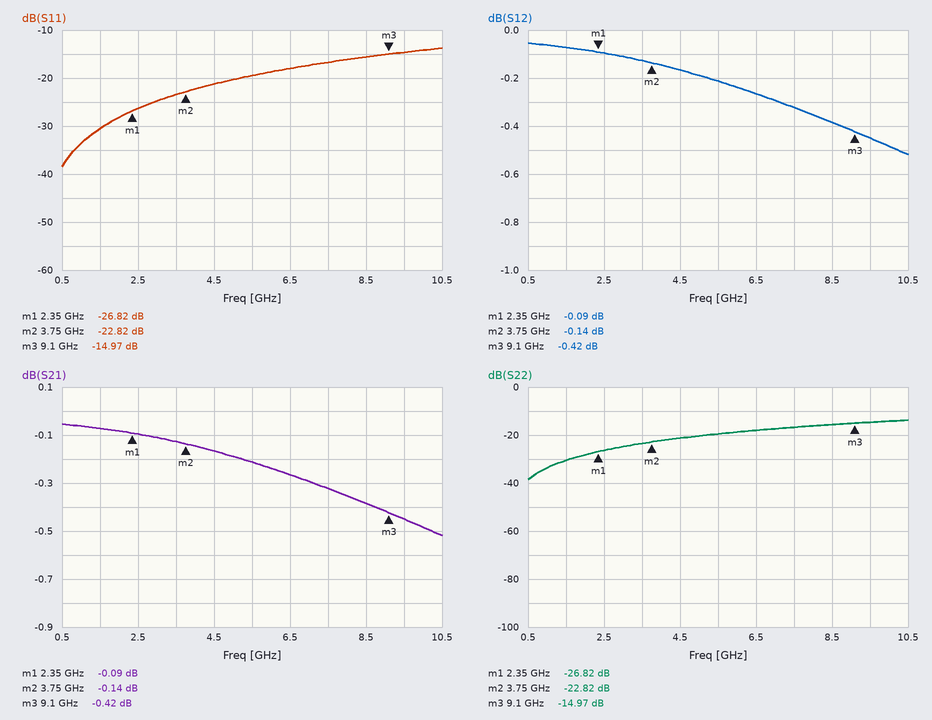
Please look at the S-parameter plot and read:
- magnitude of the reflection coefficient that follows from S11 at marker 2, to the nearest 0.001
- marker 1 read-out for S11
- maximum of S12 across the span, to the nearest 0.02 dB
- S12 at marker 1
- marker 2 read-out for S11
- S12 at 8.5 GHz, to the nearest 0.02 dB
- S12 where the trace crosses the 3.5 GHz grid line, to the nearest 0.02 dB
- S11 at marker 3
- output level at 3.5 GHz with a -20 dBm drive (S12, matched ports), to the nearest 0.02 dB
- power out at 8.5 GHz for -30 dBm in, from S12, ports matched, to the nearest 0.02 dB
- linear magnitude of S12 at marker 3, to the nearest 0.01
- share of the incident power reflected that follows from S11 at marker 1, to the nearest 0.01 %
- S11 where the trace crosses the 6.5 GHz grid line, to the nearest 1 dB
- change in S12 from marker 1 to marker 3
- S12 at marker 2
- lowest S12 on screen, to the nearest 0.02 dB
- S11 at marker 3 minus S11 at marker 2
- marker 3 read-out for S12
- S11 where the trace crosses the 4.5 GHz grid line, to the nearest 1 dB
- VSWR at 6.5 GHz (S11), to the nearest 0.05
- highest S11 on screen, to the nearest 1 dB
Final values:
0.072
-26.82 dB
-0.06 dB
-0.09 dB
-22.82 dB
-0.38 dB
-0.12 dB
-14.97 dB
-20.12 dBm
-30.38 dBm
0.95
0.21 %
-18 dB
-0.33 dB
-0.14 dB
-0.52 dB
7.85 dB
-0.42 dB
-21 dB
1.30
-14 dB
